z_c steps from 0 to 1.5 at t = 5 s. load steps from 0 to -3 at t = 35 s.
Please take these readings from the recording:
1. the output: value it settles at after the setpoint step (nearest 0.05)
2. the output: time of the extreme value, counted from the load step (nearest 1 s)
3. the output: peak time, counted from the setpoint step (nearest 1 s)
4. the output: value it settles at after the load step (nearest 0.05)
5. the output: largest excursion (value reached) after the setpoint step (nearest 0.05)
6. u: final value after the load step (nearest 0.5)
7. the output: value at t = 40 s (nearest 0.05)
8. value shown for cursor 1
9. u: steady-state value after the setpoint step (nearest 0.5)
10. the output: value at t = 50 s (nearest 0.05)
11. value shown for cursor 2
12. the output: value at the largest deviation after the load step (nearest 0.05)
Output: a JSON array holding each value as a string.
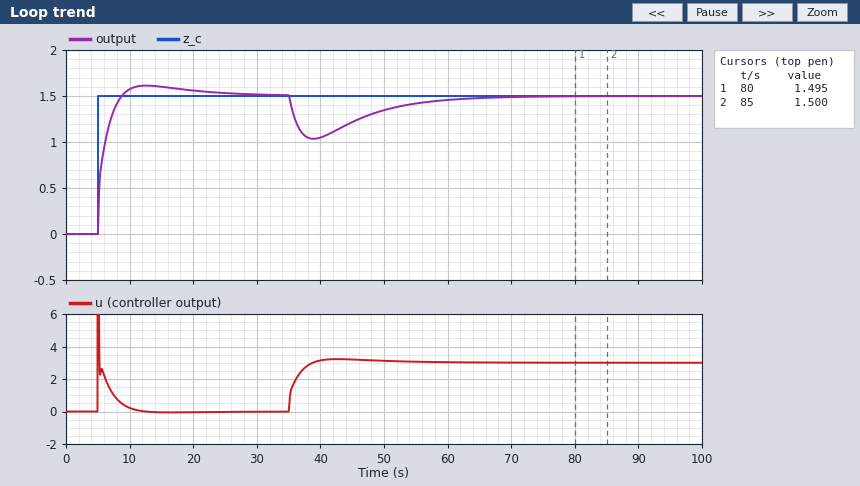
["1.50", "4 s", "8 s", "1.50", "1.60", "3.0", "1.05", "1.495", "0.0", "1.35", "1.500", "1.05"]
